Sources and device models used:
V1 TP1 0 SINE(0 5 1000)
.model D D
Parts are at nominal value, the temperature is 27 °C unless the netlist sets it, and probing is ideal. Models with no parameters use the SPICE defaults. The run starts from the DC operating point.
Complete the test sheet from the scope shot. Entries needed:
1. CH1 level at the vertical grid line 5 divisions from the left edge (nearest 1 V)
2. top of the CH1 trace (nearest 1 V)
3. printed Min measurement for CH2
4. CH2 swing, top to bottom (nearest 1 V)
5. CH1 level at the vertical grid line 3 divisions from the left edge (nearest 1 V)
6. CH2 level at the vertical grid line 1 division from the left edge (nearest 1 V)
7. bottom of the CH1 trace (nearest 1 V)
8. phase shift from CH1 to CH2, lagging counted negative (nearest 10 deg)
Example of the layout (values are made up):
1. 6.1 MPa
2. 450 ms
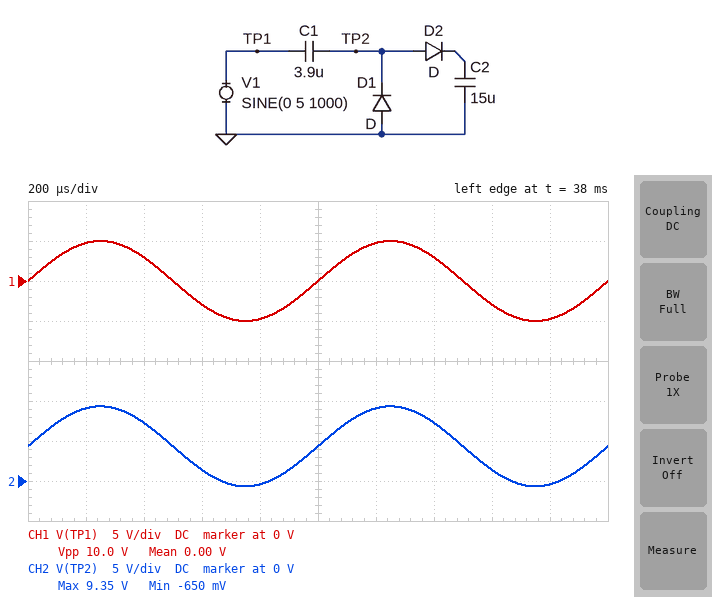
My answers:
1. 0 V
2. 5 V
3. -650 mV
4. 10 V
5. -3 V
6. 9 V
7. -5 V
8. 0 deg
